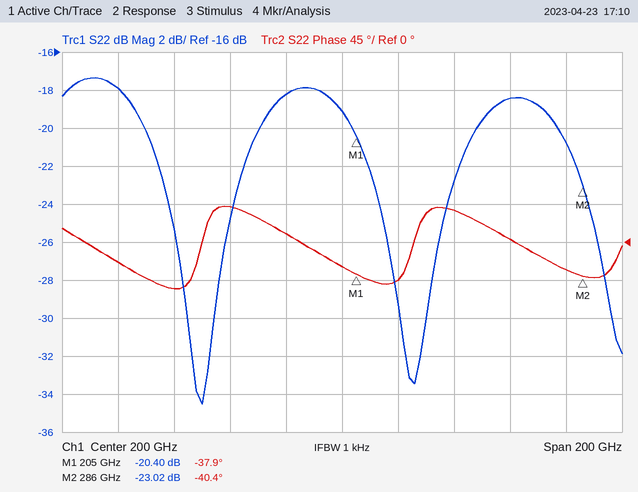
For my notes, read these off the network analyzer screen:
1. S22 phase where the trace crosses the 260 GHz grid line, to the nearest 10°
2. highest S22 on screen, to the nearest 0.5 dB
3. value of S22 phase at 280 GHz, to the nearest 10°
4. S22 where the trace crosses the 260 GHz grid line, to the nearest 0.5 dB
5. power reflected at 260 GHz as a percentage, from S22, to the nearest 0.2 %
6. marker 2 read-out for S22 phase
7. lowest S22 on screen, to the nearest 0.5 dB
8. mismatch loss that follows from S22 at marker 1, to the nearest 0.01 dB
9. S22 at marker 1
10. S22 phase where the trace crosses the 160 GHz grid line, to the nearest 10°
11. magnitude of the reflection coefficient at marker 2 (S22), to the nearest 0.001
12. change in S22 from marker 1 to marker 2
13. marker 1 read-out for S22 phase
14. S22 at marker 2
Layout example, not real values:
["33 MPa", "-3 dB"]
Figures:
["0°", "-17.5 dB", "-30°", "-18.5 dB", "1.4 %", "-40.4°", "-34.5 dB", "0.04 dB", "-20.40 dB", "40°", "0.071", "-2.62 dB", "-37.9°", "-23.02 dB"]
